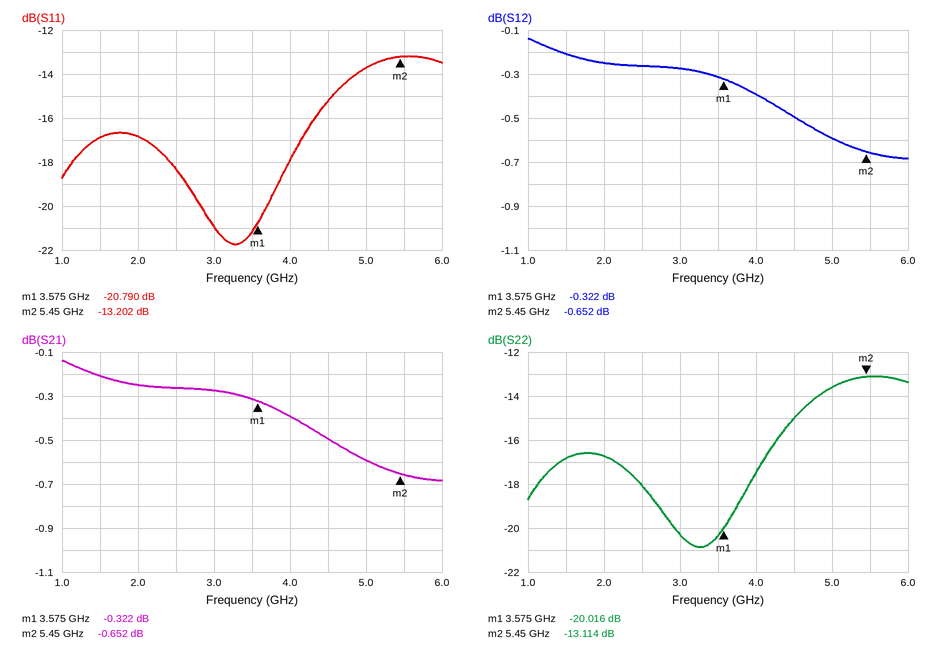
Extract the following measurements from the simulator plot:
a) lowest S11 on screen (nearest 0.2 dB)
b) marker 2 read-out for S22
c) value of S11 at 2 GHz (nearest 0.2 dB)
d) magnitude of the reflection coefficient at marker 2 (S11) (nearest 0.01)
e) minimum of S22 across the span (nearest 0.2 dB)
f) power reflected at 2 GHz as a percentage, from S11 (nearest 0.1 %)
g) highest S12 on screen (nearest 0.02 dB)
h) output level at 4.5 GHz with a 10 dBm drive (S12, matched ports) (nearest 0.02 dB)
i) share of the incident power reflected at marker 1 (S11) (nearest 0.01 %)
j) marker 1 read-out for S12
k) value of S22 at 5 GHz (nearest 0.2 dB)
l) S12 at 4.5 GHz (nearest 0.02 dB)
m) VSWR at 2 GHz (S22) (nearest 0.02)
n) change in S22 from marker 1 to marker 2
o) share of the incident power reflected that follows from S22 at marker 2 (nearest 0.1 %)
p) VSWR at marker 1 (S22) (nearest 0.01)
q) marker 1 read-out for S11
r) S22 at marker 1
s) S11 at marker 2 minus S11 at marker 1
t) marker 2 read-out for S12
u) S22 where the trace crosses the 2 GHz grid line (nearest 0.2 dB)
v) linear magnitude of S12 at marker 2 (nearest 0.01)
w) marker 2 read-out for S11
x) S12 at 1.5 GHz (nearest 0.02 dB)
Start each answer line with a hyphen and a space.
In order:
- -21.8 dB
- -13.114 dB
- -16.8 dB
- 0.22
- -20.8 dB
- 2.1 %
- -0.14 dB
- 9.50 dBm
- 0.83 %
- -0.322 dB
- -13.6 dB
- -0.50 dB
- 1.34
- 6.902 dB
- 4.9 %
- 1.22
- -20.790 dB
- -20.016 dB
- 7.588 dB
- -0.652 dB
- -16.8 dB
- 0.93
- -13.202 dB
- -0.20 dB
